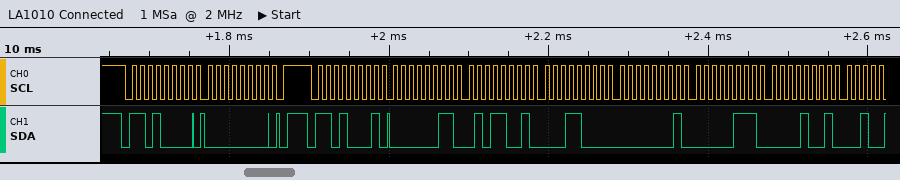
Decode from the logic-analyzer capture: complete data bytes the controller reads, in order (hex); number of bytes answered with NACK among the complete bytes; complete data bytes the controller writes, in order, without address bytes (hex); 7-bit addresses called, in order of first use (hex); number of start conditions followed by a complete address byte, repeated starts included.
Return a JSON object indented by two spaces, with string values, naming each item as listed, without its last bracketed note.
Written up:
{
  "complete data bytes the controller reads, in order": "03 59 18 01 07 09",
  "number of bytes answered with NACK among the complete bytes": "0",
  "complete data bytes the controller writes, in order, without address bytes": "00",
  "7-bit addresses called, in order of first use": "0x68",
  "number of start conditions followed by a complete address byte, repeated starts included": "2"
}
